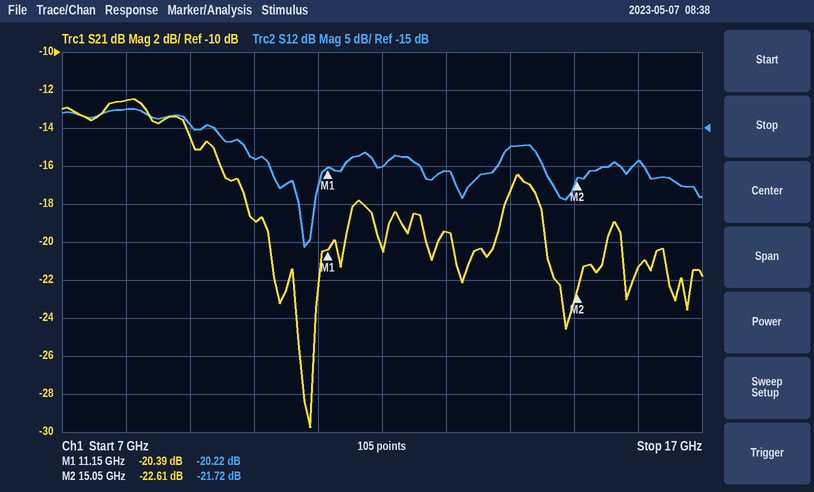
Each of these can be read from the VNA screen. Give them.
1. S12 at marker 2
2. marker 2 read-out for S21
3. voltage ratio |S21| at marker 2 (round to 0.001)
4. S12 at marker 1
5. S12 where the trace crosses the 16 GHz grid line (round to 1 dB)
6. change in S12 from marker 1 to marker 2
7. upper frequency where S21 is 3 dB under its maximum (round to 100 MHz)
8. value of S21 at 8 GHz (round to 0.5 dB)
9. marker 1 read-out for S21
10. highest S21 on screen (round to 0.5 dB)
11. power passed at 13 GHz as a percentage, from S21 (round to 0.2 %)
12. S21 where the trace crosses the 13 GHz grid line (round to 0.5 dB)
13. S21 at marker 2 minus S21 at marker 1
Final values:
-21.72 dB
-22.61 dB
0.074
-20.22 dB
-19 dB
-1.50 dB
9.4 GHz
-12.5 dB
-20.39 dB
-12.5 dB
1.2 %
-19.5 dB
-2.22 dB
